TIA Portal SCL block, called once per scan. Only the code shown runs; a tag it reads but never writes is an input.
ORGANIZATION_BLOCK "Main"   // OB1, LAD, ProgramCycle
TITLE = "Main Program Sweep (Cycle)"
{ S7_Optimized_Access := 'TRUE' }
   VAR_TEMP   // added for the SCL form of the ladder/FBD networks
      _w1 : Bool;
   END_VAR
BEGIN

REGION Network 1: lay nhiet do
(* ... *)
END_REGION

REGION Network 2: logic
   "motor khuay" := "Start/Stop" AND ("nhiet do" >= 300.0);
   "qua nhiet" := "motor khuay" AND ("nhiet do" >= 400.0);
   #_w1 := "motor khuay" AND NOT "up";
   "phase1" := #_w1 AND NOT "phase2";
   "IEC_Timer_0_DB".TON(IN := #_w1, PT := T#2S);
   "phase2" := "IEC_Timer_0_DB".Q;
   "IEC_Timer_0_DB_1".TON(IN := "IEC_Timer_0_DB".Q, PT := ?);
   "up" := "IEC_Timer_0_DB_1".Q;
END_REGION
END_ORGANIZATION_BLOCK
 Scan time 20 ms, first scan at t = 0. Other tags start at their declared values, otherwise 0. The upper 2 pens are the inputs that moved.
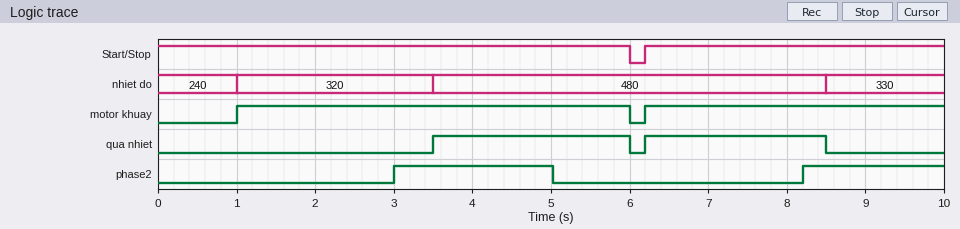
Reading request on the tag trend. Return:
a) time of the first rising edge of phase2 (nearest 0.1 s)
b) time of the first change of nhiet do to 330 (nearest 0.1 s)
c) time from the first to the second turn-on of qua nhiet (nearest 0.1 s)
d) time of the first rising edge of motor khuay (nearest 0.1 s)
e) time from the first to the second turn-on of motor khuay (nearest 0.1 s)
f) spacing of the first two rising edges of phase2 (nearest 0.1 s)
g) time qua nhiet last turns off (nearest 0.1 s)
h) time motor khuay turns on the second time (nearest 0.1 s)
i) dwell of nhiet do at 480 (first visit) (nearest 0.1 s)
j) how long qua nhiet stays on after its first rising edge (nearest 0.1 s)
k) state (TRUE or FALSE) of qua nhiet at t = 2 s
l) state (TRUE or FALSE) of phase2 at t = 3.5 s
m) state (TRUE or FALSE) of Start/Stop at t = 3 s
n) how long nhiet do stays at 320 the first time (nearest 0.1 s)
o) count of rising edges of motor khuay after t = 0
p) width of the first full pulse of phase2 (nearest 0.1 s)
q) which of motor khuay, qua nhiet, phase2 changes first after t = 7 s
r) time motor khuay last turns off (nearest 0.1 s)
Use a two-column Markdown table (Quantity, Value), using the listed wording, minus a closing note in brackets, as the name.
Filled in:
| Quantity | Value |
|---|---|
| time of the first rising edge of phase2 | 3.0 s |
| time of the first change of nhiet do to 330 | 8.5 s |
| time from the first to the second turn-on of qua nhiet | 2.7 s |
| time of the first rising edge of motor khuay | 1.0 s |
| time from the first to the second turn-on of motor khuay | 5.2 s |
| spacing of the first two rising edges of phase2 | 5.2 s |
| time qua nhiet last turns off | 8.5 s |
| time motor khuay turns on the second time | 6.2 s |
| dwell of nhiet do at 480 (first visit) | 5.0 s |
| how long qua nhiet stays on after its first rising edge | 2.5 s |
| state (TRUE or FALSE) of qua nhiet at t = 2 s | FALSE |
| state (TRUE or FALSE) of phase2 at t = 3.5 s | TRUE |
| state (TRUE or FALSE) of Start/Stop at t = 3 s | TRUE |
| how long nhiet do stays at 320 the first time | 2.5 s |
| count of rising edges of motor khuay after t = 0 | 2 |
| width of the first full pulse of phase2 | 2.0 s |
| which of motor khuay, qua nhiet, phase2 changes first after t = 7 s | phase2 |
| time motor khuay last turns off | 6.0 s |
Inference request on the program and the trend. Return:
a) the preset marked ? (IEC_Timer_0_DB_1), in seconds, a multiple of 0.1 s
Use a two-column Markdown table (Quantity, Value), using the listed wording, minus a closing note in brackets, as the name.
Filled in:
| Quantity | Value |
|---|---|
| the preset marked ? (IEC_Timer_0_DB_1), in seconds, a multiple of 0.1 s | 2.0 s |
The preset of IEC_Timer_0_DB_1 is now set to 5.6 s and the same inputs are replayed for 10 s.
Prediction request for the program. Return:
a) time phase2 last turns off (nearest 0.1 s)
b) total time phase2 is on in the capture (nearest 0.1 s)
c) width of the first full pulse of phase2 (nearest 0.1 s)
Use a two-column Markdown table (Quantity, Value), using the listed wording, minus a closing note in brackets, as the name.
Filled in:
| Quantity | Value |
|---|---|
| time phase2 last turns off | 6.0 s |
| total time phase2 is on in the capture | 4.8 s |
| width of the first full pulse of phase2 | 3.0 s |
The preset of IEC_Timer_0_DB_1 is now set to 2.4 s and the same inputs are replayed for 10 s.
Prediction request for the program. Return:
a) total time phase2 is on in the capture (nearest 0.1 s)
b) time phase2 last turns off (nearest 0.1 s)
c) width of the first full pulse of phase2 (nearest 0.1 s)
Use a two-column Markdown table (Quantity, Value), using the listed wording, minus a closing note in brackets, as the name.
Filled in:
| Quantity | Value |
|---|---|
| total time phase2 is on in the capture | 4.2 s |
| time phase2 last turns off | 5.4 s |
| width of the first full pulse of phase2 | 2.4 s |
